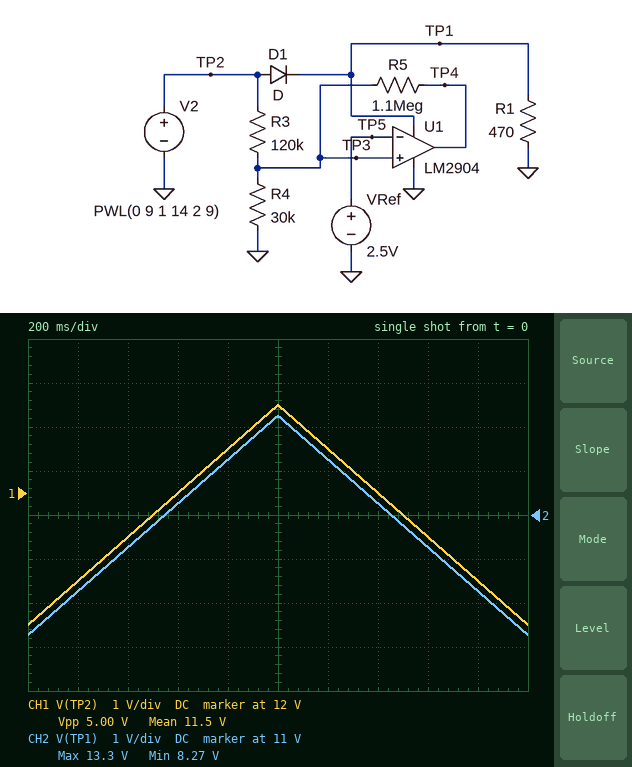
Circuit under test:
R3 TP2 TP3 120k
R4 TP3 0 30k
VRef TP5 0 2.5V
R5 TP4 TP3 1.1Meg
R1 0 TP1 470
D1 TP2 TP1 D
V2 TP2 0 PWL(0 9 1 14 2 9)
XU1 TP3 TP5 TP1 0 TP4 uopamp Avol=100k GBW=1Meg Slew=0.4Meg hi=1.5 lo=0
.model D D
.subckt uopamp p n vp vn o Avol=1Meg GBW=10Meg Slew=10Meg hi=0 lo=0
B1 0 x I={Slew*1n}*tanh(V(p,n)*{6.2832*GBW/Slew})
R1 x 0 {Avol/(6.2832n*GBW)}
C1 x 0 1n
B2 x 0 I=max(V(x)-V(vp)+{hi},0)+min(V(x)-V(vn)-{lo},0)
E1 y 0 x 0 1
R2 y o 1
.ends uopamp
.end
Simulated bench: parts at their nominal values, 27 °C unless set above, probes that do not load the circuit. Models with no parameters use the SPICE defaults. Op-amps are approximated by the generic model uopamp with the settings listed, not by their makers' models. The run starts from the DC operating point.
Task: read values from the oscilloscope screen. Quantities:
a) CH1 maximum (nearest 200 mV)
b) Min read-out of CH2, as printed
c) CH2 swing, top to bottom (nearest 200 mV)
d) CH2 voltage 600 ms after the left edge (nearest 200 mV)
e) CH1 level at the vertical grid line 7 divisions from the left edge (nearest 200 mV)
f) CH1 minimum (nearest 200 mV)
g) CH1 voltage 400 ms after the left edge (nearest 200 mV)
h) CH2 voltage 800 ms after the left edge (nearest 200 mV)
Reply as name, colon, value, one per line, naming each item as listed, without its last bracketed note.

CH1 maximum: 14.0 V
Min read-out of CH2, as printed: 8.27 V
CH2 swing, top to bottom: 5.0 V
CH2 voltage 600 ms after the left edge: 11.2 V
CH1 level at the vertical grid line 7 divisions from the left edge: 12.0 V
CH1 minimum: 9.0 V
CH1 voltage 400 ms after the left edge: 11.0 V
CH2 voltage 800 ms after the left edge: 12.2 V
